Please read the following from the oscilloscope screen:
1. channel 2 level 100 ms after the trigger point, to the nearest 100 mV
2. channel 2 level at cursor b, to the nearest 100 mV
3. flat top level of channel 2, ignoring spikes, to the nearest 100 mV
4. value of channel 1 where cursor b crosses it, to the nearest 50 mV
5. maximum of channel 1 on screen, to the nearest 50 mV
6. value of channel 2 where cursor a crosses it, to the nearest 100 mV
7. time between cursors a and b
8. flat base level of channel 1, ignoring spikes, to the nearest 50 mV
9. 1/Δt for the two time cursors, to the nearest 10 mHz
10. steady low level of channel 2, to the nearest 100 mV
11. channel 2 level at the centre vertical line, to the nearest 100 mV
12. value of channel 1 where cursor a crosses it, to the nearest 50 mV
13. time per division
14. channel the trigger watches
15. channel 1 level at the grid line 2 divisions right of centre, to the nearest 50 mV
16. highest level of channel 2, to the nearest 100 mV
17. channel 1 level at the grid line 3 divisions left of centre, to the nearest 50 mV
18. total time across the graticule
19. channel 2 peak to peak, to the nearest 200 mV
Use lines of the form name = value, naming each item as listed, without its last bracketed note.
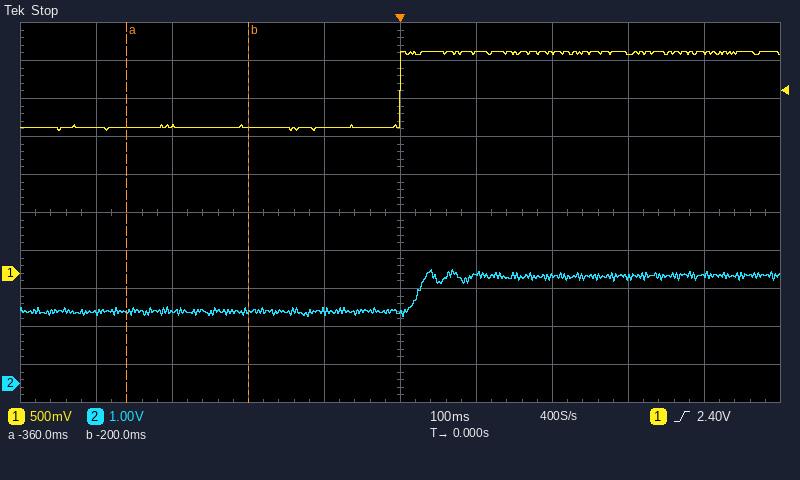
channel 2 level 100 ms after the trigger point, to the nearest 100 mV = 2.9 V
channel 2 level at cursor b, to the nearest 100 mV = 1.9 V
flat top level of channel 2, ignoring spikes, to the nearest 100 mV = 2.8 V
value of channel 1 where cursor b crosses it, to the nearest 50 mV = 1.90 V
maximum of channel 1 on screen, to the nearest 50 mV = 2.90 V
value of channel 2 where cursor a crosses it, to the nearest 100 mV = 1.9 V
time between cursors a and b = 160 ms
flat base level of channel 1, ignoring spikes, to the nearest 50 mV = 1.90 V
1/Δt for the two time cursors, to the nearest 10 mHz = 6.25 Hz
steady low level of channel 2, to the nearest 100 mV = 1.9 V
channel 2 level at the centre vertical line, to the nearest 100 mV = 1.8 V
value of channel 1 where cursor a crosses it, to the nearest 50 mV = 1.90 V
time per division = 100 ms
channel the trigger watches = channel 1
channel 1 level at the grid line 2 divisions right of centre, to the nearest 50 mV = 2.90 V
highest level of channel 2, to the nearest 100 mV = 3.0 V
channel 1 level at the grid line 3 divisions left of centre, to the nearest 50 mV = 1.95 V
total time across the graticule = 1 s
channel 2 peak to peak, to the nearest 200 mV = 1.2 V
